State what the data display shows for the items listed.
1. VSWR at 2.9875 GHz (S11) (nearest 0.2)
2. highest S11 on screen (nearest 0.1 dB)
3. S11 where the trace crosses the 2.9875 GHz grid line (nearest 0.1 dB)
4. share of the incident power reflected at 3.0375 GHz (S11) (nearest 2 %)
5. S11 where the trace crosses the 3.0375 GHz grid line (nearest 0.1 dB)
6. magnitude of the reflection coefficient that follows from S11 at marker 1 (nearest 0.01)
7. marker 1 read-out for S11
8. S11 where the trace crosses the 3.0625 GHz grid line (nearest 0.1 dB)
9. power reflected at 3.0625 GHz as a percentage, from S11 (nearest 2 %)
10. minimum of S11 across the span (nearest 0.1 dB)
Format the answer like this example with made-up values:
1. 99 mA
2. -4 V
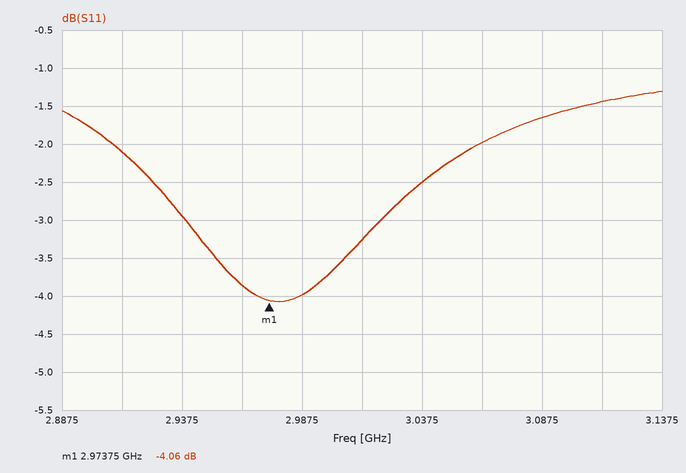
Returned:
1. 4.4
2. -1.3 dB
3. -4.0 dB
4. 56 %
5. -2.5 dB
6. 0.63
7. -4.06 dB
8. -2.0 dB
9. 64 %
10. -4.1 dB
